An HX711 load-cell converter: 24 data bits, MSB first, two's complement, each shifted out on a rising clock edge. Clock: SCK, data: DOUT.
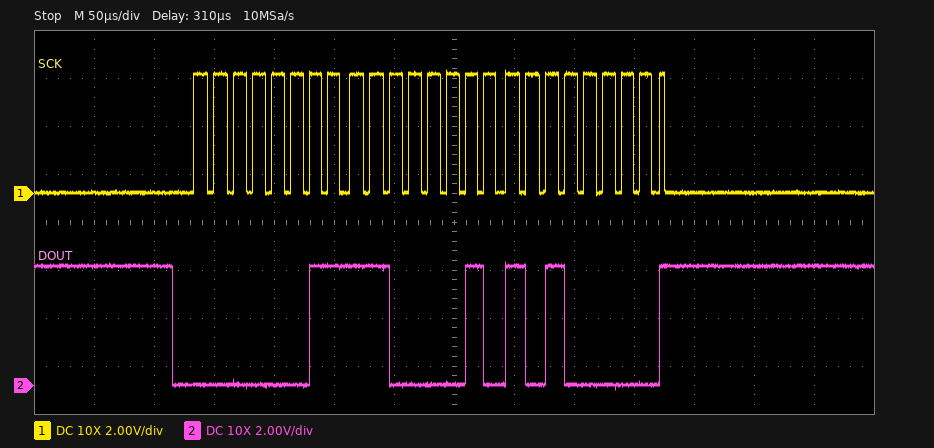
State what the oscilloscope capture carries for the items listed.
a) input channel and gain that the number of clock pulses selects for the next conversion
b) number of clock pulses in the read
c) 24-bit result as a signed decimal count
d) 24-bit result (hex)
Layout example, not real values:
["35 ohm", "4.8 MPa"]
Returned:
["channel A, gain 128", "25", "246432", "0x03C2A0"]
